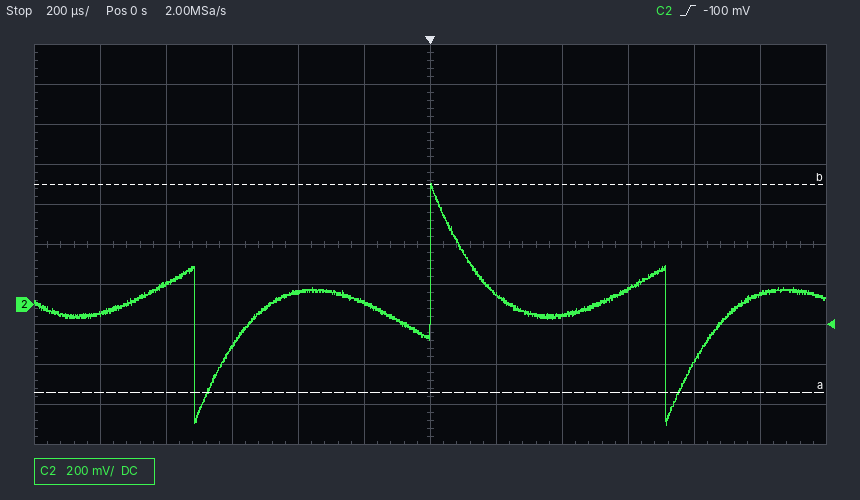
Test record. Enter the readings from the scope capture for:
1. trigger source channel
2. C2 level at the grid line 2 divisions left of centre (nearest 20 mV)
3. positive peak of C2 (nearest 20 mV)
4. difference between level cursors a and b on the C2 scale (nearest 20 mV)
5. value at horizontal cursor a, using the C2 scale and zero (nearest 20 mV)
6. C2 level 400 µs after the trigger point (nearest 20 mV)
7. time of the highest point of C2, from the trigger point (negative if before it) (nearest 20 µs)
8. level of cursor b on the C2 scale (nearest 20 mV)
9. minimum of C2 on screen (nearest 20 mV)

C2
60 mV
600 mV
1.04 V
-440 mV
-60 mV
0 µs
600 mV
-600 mV
